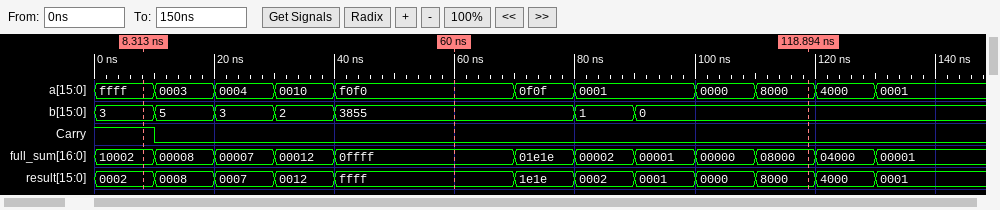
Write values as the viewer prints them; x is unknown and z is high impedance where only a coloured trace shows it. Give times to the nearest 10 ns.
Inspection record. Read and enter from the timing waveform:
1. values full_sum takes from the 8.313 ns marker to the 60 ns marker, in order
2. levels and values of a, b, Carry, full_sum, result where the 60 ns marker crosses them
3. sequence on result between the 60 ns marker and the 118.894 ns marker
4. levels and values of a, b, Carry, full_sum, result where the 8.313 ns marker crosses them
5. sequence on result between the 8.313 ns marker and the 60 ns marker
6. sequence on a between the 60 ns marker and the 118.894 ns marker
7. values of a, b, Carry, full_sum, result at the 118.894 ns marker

10002, 00008, 00007, 00012, 0ffff
a=f0f0, b=3855, Carry=0, full_sum=0ffff, result=ffff
ffff, 1e1e, 0002, 0001, 0000, 8000
a=ffff, b=3, Carry=1, full_sum=10002, result=0002
0002, 0008, 0007, 0012, ffff
f0f0, 0f0f, 0001, 0000, 8000
a=8000, b=0, Carry=0, full_sum=08000, result=8000
